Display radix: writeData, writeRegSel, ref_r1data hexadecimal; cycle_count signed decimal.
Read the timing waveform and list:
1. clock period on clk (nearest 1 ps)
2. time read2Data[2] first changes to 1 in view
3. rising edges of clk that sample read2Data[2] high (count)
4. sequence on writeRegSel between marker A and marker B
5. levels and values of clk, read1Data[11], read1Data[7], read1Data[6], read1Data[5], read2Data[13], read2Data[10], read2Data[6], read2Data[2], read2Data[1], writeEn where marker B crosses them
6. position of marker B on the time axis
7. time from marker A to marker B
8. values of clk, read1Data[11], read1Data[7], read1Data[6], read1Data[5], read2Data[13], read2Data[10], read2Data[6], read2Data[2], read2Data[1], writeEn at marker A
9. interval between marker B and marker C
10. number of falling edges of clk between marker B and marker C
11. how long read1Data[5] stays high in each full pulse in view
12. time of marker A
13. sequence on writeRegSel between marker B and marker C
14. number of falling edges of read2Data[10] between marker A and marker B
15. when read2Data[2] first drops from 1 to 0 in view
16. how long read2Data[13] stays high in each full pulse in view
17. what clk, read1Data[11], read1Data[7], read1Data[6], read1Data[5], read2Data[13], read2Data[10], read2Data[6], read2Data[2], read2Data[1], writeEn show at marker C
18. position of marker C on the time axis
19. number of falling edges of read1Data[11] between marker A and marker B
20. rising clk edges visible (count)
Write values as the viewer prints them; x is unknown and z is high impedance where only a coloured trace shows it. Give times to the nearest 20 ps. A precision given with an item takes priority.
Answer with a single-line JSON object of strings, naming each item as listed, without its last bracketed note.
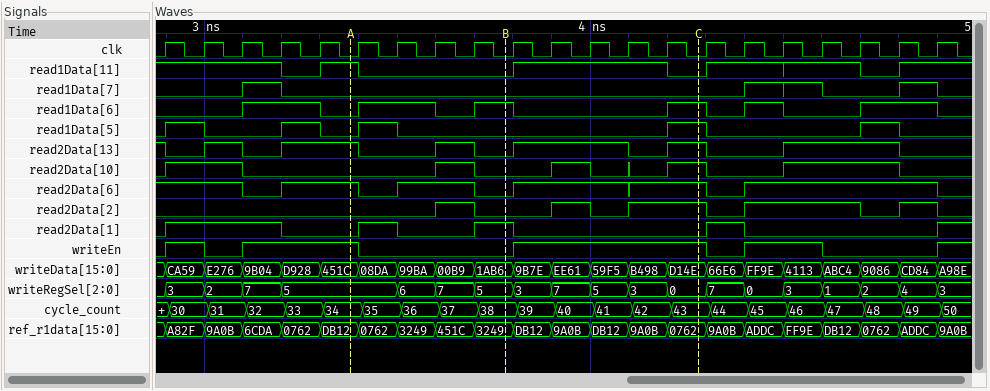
{"clock period on clk": "100 ps", "time read2Data[2] first changes to 1 in view": "3600 ps", "rising edges of clk that sample read2Data[2] high": "8", "sequence on writeRegSel between marker A and marker B": "5, 6, 7, 5", "levels and values of clk, read1Data[11], read1Data[7], read1Data[6], read1Data[5], read2Data[13], read2Data[10], read2Data[6], read2Data[2], read2Data[1], writeEn where marker B crosses them": "clk=0, read1Data[11]=0, read1Data[7]=0, read1Data[6]=1, read1Data[5]=0, read2Data[13]=0, read2Data[10]=0, read2Data[6]=0, read2Data[2]=0, read2Data[1]=1, writeEn=0", "position of marker B on the time axis": "3780 ps", "time from marker A to marker B": "400 ps", "values of clk, read1Data[11], read1Data[7], read1Data[6], read1Data[5], read2Data[13], read2Data[10], read2Data[6], read2Data[2], read2Data[1], writeEn at marker A": "clk=0, read1Data[11]=1, read1Data[7]=0, read1Data[6]=0, read1Data[5]=0, read2Data[13]=1, read2Data[10]=0, read2Data[6]=1, read2Data[2]=0, read2Data[1]=0, writeEn=1", "interval between marker B and marker C": "500 ps", "number of falling edges of clk between marker B and marker C": "5", "how long read1Data[5] stays high in each full pulse in view": "100 ps, 100 ps, 100 ps, 100 ps, 100 ps", "time of marker A": "3380 ps", "sequence on writeRegSel between marker B and marker C": "5, 3, 7, 5, 3, 0", "number of falling edges of read2Data[10] between marker A and marker B": "1", "when read2Data[2] first drops from 1 to 0 in view": "3700 ps", "how long read2Data[13] stays high in each full pulse in view": "100 ps, 200 ps, 100 ps, 300 ps, 100 ps, 300 ps", "what clk, read1Data[11], read1Data[7], read1Data[6], read1Data[5], read2Data[13], read2Data[10], read2Data[6], read2Data[2], read2Data[1], writeEn show at marker C": "clk=0, read1Data[11]=0, read1Data[7]=0, read1Data[6]=1, read1Data[5]=1, read2Data[13]=1, read2Data[10]=1, read2Data[6]=1, read2Data[2]=1, read2Data[1]=0, writeEn=1", "position of marker C on the time axis": "4280 ps", "number of falling edges of read1Data[11] between marker A and marker B": "1", "rising clk edges visible": "21"}
